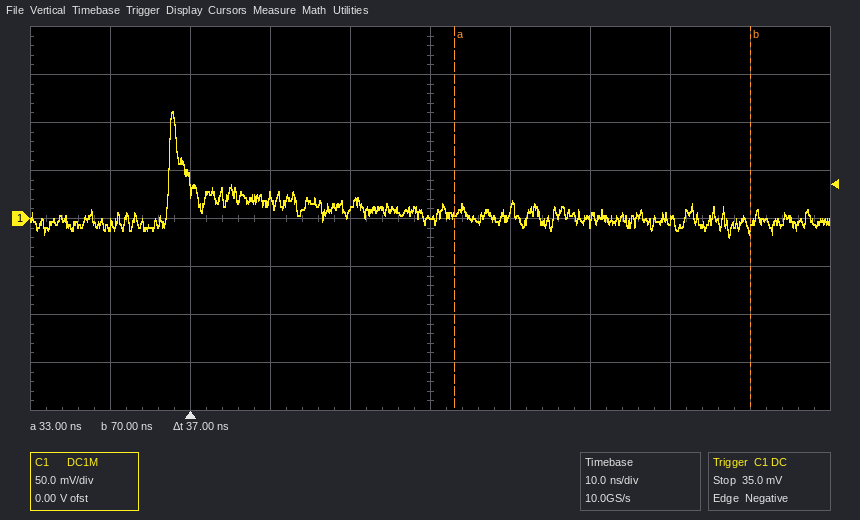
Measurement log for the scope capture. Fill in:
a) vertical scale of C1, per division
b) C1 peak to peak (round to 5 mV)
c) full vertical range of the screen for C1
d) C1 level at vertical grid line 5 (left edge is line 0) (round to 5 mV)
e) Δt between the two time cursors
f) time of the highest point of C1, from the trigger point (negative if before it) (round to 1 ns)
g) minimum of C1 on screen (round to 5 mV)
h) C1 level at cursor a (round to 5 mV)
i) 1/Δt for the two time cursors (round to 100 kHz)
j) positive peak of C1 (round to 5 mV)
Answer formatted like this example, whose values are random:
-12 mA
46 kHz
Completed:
50 mV
130 mV
400 mV
0 mV
37 ns
-2 ns
-20 mV
5 mV
27.0 MHz
110 mV
